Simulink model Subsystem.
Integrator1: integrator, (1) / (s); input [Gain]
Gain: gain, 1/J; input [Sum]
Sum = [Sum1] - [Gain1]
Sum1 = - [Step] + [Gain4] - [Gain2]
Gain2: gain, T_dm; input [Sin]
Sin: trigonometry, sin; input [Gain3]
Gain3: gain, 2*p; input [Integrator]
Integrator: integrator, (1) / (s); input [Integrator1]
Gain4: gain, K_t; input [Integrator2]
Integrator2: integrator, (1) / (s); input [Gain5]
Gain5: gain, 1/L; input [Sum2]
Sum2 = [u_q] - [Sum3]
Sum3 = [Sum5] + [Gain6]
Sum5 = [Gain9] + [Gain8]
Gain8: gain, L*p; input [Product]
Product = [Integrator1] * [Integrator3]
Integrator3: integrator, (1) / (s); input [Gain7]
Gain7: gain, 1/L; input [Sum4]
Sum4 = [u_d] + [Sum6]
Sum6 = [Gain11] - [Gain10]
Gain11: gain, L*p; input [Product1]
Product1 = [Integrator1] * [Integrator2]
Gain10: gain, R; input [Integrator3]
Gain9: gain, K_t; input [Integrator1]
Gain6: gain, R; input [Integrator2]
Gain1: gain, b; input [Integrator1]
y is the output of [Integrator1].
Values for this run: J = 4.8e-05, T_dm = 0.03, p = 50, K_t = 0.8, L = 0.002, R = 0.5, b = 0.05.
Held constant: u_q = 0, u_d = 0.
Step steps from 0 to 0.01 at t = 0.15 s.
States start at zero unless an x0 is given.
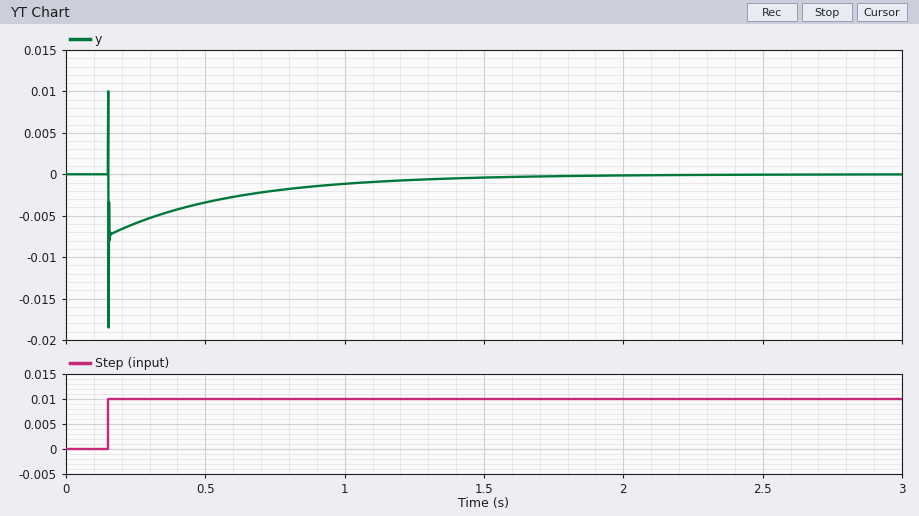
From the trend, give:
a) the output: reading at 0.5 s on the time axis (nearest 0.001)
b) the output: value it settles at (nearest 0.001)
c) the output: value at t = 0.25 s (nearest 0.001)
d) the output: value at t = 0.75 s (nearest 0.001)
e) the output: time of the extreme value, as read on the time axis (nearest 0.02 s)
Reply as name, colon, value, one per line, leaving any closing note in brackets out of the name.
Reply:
the output: reading at 0.5 s on the time axis: -0.003
the output: value it settles at: 0.000
the output: value at t = 0.25 s: -0.006
the output: value at t = 0.75 s: -0.002
the output: time of the extreme value, as read on the time axis: 0.16 s
